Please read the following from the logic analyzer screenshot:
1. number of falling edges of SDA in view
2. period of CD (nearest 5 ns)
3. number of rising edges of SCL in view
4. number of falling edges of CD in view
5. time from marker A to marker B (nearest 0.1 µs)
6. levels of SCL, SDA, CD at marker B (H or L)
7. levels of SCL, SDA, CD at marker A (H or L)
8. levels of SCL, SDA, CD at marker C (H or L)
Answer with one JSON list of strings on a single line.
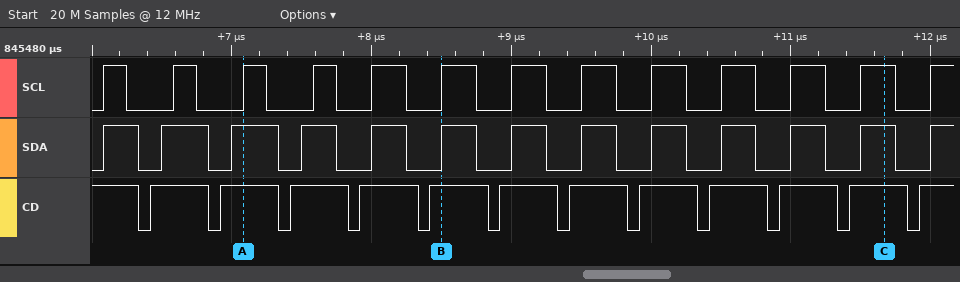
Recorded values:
["12", "500 ns", "13", "12", "1.4 µs", "SCL=H, SDA=H, CD=H", "SCL=H, SDA=H, CD=H", "SCL=H, SDA=H, CD=H"]
